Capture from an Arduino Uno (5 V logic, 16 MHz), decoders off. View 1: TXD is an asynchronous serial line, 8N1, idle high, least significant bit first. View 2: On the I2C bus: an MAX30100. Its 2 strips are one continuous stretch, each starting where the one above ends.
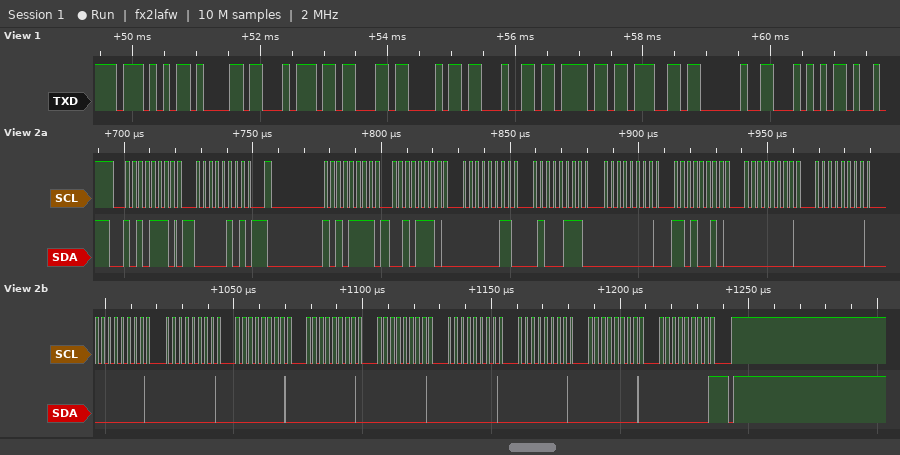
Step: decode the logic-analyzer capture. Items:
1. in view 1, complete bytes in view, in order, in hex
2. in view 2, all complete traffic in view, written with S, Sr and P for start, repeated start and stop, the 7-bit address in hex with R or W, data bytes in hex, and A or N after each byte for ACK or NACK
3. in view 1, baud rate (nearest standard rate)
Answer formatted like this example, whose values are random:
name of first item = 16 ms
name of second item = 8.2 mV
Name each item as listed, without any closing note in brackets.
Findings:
in view 1, complete bytes in view, in order, in hex = 0x57 0x61 0x74 0x63 0x68 0x64 0x6F 0x67 0x20 0x54
in view 2, all complete traffic in view, written with S, Sr and P for start, repeated start and stop, the 7-bit address in hex with R or W, data bytes in hex, and A or N after each byte for ACK or NACK = S 57W A 05 A Sr 57R A 2E A 03 A 47 A 00 A D2 A 00 A 00 A 00 A 00 A 00 A 00 A 00 A 00 A 00 A 00 A 00 N P
in view 1, baud rate = 9600 baud
